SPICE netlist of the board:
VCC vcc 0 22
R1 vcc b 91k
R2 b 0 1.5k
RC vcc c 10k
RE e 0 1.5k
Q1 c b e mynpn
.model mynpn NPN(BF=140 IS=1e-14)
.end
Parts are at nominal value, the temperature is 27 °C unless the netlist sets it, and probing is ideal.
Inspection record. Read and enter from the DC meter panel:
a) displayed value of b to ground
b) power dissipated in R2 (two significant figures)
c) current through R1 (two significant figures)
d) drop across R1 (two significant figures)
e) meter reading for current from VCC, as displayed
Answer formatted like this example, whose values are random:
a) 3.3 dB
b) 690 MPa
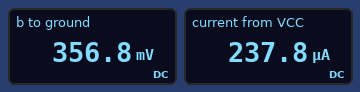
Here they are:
a) 356.8 mV
b) 85 µW
c) 240 µA
d) 22 V
e) 237.8 µA
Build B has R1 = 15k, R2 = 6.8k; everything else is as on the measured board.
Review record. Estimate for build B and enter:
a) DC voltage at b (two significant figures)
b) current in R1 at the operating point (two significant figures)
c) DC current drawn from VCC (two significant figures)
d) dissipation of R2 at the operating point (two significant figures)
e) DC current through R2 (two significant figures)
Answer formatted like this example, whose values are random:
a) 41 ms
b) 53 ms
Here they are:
a) 4.3 V
b) 1.2 mA
c) 3.0 mA
d) 2.7 mW
e) 630 µA
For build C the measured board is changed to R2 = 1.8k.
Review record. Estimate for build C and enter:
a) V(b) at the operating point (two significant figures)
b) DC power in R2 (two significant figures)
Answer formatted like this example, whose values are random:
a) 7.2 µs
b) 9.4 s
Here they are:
a) 430 mV
b) 100 µW
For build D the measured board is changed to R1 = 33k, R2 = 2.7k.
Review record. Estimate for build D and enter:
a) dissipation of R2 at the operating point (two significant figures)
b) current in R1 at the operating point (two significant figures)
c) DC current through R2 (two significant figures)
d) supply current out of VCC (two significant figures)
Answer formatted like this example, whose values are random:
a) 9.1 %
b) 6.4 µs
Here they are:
a) 1.0 mW
b) 620 µA
c) 610 µA
d) 1.3 mA
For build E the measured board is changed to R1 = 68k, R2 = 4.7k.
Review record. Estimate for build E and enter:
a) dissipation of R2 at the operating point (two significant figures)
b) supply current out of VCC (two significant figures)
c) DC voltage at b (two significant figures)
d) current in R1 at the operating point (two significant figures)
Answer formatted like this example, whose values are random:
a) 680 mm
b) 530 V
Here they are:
a) 420 µW
b) 810 µA
c) 1.4 V
d) 300 µA
